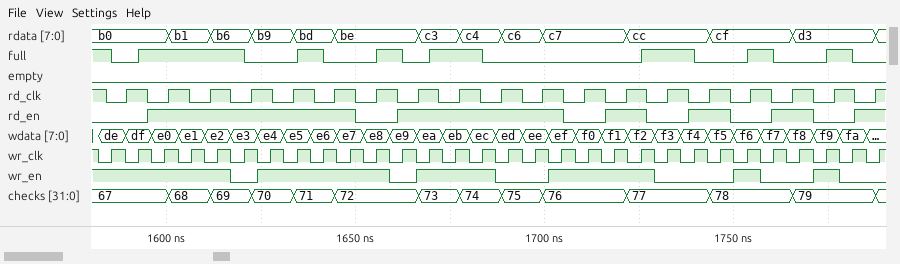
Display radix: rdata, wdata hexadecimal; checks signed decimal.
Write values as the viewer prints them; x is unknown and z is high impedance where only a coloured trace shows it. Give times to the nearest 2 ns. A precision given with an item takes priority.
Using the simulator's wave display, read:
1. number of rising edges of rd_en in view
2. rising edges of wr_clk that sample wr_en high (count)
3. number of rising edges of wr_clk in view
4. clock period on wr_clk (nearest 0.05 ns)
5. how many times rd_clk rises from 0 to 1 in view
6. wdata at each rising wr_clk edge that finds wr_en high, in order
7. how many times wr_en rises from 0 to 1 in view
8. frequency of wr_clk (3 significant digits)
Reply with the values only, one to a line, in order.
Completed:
6
19
30
7 ns
19
de, df, e0, e1, e2, e4, e5, e6, e7, e8, ea, eb, ec, ef, f0, f1, f2, f6, f9
5
143 MHz
